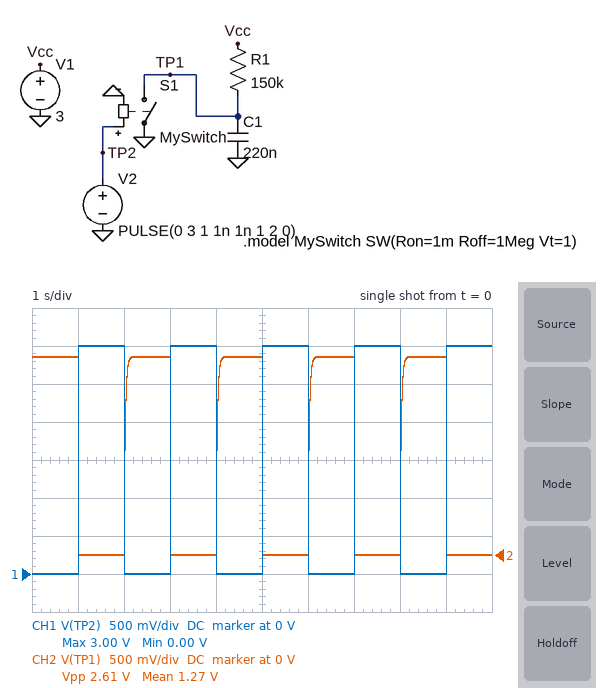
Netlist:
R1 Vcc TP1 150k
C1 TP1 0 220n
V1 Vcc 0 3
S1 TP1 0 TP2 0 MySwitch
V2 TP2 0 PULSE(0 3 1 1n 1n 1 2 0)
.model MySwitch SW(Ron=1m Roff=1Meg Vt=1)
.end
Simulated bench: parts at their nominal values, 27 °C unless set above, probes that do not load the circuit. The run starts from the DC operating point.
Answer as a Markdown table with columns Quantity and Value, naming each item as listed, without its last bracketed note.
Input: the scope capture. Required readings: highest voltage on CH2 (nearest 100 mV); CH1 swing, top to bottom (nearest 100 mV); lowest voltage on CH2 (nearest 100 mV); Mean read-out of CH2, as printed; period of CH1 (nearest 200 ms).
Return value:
| Quantity | Value |
|---|---|
| highest voltage on CH2 | 2.6 V |
| CH1 swing, top to bottom | 3.0 V |
| lowest voltage on CH2 | 0 V |
| Mean read-out of CH2, as printed | 1.27 V |
| period of CH1 | 2.0 s |
